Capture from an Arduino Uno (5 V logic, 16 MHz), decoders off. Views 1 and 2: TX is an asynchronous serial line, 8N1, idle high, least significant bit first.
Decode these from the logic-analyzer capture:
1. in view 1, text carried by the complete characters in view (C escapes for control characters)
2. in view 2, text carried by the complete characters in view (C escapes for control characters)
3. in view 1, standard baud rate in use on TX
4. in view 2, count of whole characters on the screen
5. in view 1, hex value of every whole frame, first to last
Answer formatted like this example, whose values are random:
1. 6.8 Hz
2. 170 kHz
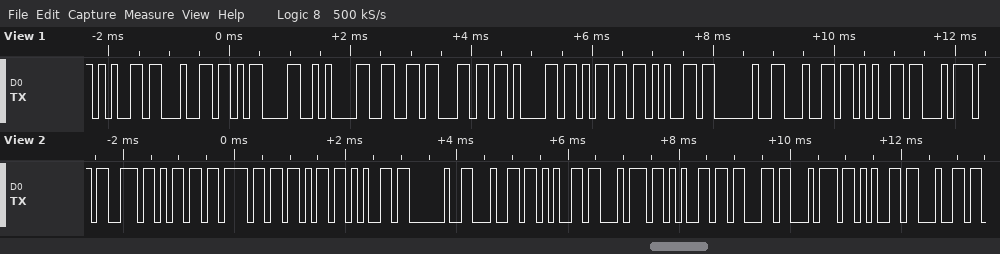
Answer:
1. "ed\r\nflame det"
2. "smoke detected"
3. 9600 baud
4. 14
5. 65 64 0D 0A 66 6C 61 6D 65 20 64 65 74
